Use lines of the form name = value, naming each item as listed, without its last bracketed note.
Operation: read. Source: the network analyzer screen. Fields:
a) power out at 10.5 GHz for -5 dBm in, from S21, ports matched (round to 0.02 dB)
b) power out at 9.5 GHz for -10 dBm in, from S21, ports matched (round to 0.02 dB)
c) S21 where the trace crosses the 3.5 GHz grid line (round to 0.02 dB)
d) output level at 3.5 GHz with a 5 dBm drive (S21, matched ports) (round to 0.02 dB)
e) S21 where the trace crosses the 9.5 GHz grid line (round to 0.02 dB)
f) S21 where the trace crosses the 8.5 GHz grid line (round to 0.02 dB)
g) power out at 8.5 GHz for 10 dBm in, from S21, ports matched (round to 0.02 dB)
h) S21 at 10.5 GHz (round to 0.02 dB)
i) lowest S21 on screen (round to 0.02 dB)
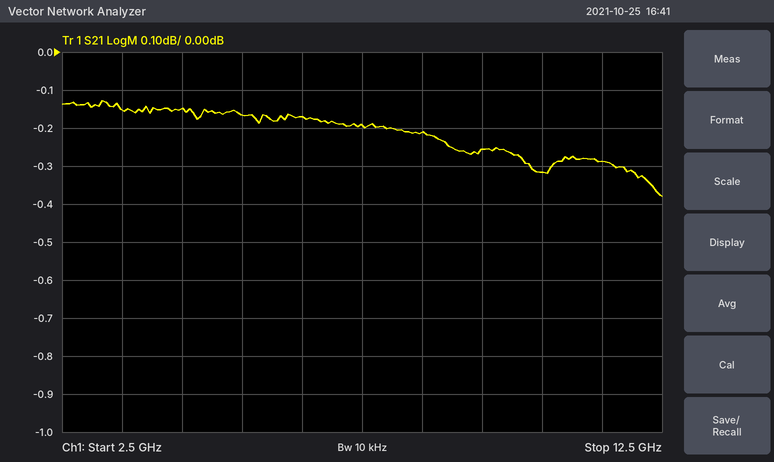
power out at 10.5 GHz for -5 dBm in, from S21, ports matched = -5.32 dBm
power out at 9.5 GHz for -10 dBm in, from S21, ports matched = -10.26 dBm
S21 where the trace crosses the 3.5 GHz grid line = -0.16 dB
output level at 3.5 GHz with a 5 dBm drive (S21, matched ports) = 4.84 dBm
S21 where the trace crosses the 9.5 GHz grid line = -0.26 dB
S21 where the trace crosses the 8.5 GHz grid line = -0.22 dB
power out at 8.5 GHz for 10 dBm in, from S21, ports matched = 9.78 dBm
S21 at 10.5 GHz = -0.32 dB
lowest S21 on screen = -0.38 dB
